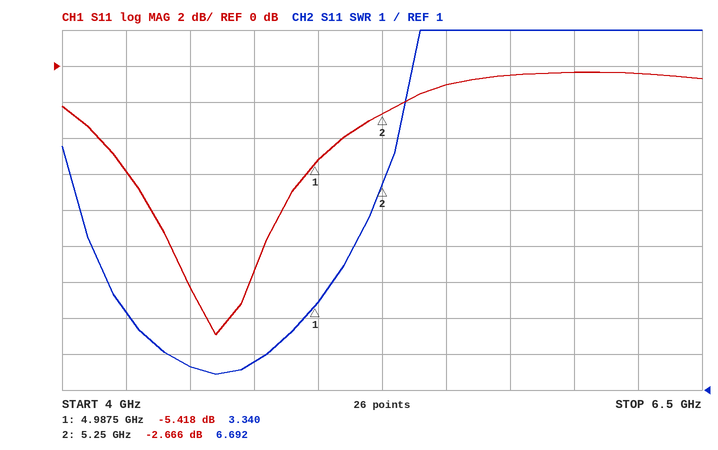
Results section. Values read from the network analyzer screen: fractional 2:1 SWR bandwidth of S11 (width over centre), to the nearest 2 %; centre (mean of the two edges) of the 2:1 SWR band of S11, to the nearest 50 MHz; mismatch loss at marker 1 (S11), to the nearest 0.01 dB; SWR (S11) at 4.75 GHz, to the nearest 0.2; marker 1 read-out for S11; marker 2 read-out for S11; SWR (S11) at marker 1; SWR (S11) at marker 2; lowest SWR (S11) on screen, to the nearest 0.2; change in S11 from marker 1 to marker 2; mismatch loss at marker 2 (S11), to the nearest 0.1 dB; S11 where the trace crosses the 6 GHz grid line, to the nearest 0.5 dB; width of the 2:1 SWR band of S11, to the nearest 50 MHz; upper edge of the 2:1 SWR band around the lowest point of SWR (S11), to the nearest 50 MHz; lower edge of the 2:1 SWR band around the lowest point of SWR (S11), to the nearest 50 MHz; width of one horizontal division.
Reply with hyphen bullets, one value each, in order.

- 8 %
- 4.60 GHz
- 1.47 dB
- 1.8
- -5.418 dB
- -2.666 dB
- 3.340
- 6.692
- 1.4
- 2.752 dB
- 3.4 dB
- -0.5 dB
- 400 MHz
- 4.80 GHz
- 4.40 GHz
- 250 MHz
